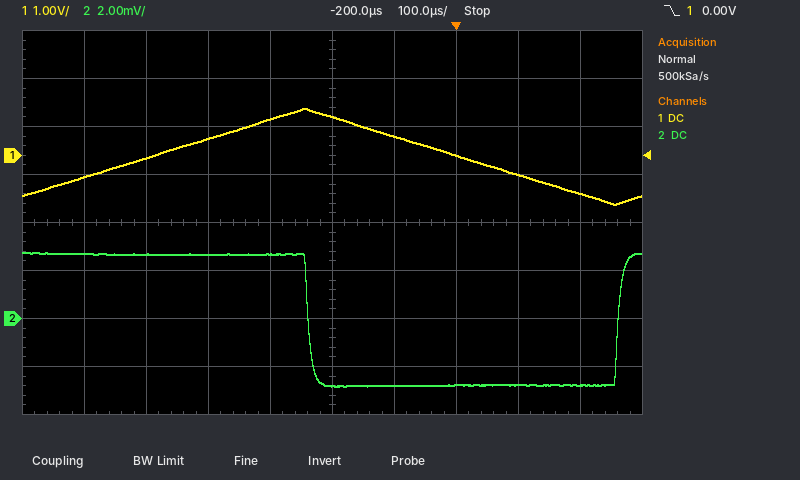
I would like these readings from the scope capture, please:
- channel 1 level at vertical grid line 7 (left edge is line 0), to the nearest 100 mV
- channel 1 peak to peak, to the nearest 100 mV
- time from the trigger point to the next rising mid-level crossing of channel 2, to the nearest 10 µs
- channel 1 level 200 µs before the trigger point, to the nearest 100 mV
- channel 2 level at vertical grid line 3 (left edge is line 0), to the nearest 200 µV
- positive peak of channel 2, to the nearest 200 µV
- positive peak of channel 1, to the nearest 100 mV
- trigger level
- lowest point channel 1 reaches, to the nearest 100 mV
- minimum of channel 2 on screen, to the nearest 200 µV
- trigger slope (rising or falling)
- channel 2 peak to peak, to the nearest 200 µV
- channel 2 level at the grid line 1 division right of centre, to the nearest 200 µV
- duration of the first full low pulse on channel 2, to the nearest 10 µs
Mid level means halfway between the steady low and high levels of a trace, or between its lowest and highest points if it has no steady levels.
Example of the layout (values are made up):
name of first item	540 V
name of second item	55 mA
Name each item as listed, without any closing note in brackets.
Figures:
channel 1 level at vertical grid line 7 (left edge is line 0), to the nearest 100 mV	0.0 V
channel 1 peak to peak, to the nearest 100 mV	2.0 V
time from the trigger point to the next rising mid-level crossing of channel 2, to the nearest 10 µs	260 µs
channel 1 level 200 µs before the trigger point, to the nearest 100 mV	800 mV
channel 2 level at vertical grid line 3 (left edge is line 0), to the nearest 200 µV	2.6 mV
positive peak of channel 2, to the nearest 200 µV	2.8 mV
positive peak of channel 1, to the nearest 100 mV	1.0 V
trigger level	0.00 V
lowest point channel 1 reaches, to the nearest 100 mV	-1.0 V
minimum of channel 2 on screen, to the nearest 200 µV	-2.8 mV
trigger slope	falling
channel 2 peak to peak, to the nearest 200 µV	5.6 mV
channel 2 level at the grid line 1 division right of centre, to the nearest 200 µV	-2.8 mV
duration of the first full low pulse on channel 2, to the nearest 10 µs	500 µs
